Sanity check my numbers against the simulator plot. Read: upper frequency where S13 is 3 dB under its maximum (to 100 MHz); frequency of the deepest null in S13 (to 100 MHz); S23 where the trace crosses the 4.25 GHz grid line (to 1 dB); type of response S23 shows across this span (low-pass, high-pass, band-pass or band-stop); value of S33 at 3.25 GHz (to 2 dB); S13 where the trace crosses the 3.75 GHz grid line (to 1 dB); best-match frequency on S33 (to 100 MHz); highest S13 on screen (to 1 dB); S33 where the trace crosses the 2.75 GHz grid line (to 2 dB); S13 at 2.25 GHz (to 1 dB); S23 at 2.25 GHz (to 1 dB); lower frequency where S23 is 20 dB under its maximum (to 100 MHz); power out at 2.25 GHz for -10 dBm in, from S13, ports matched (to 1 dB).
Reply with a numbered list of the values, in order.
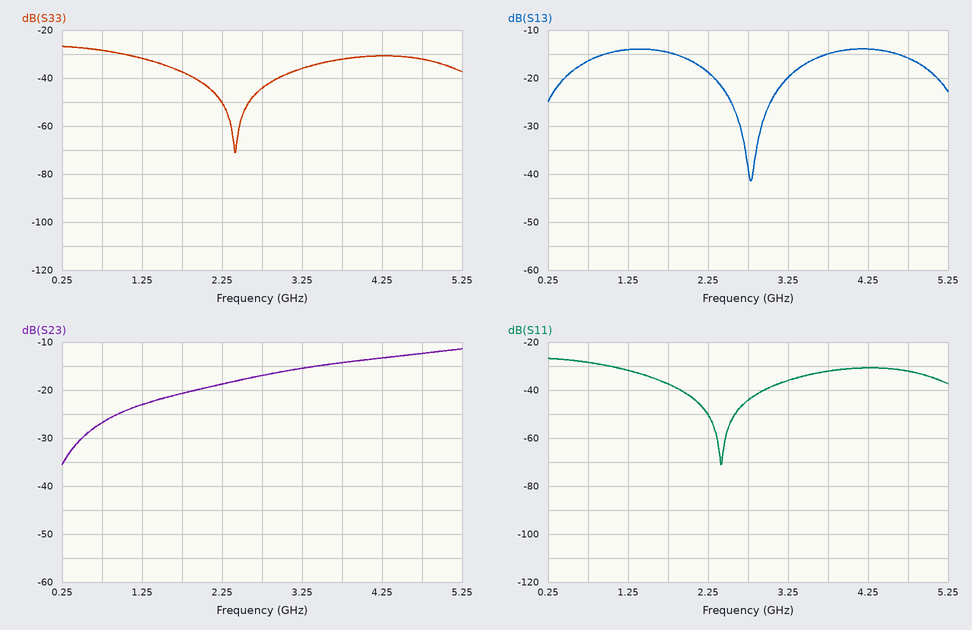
1. 4.9 GHz
2. 2.8 GHz
3. -13 dB
4. high-pass
5. -36 dB
6. -15 dB
7. 2.4 GHz
8. -14 dB
9. -44 dB
10. -19 dB
11. -19 dB
12. 400 MHz
13. -29 dBm
